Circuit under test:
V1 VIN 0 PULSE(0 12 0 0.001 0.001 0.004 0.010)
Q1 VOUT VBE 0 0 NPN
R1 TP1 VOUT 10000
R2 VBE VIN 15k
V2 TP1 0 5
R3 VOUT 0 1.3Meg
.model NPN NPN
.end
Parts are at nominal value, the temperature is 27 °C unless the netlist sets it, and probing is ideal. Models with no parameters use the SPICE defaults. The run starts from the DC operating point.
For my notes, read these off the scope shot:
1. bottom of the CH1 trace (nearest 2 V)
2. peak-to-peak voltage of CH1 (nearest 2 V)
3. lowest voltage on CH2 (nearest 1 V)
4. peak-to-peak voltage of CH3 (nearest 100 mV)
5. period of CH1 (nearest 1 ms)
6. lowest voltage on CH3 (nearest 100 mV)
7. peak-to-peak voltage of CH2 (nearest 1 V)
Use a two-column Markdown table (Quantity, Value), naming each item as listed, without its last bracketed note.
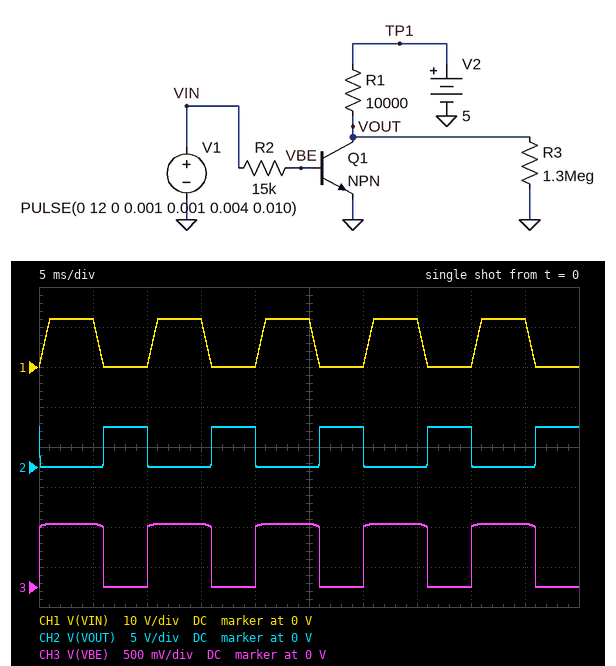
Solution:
| Quantity | Value |
|---|---|
| bottom of the CH1 trace | 0 V |
| peak-to-peak voltage of CH1 | 12 V |
| lowest voltage on CH2 | 0 V |
| peak-to-peak voltage of CH3 | 800 mV |
| period of CH1 | 10 ms |
| lowest voltage on CH3 | 0 V |
| peak-to-peak voltage of CH2 | 5 V |
